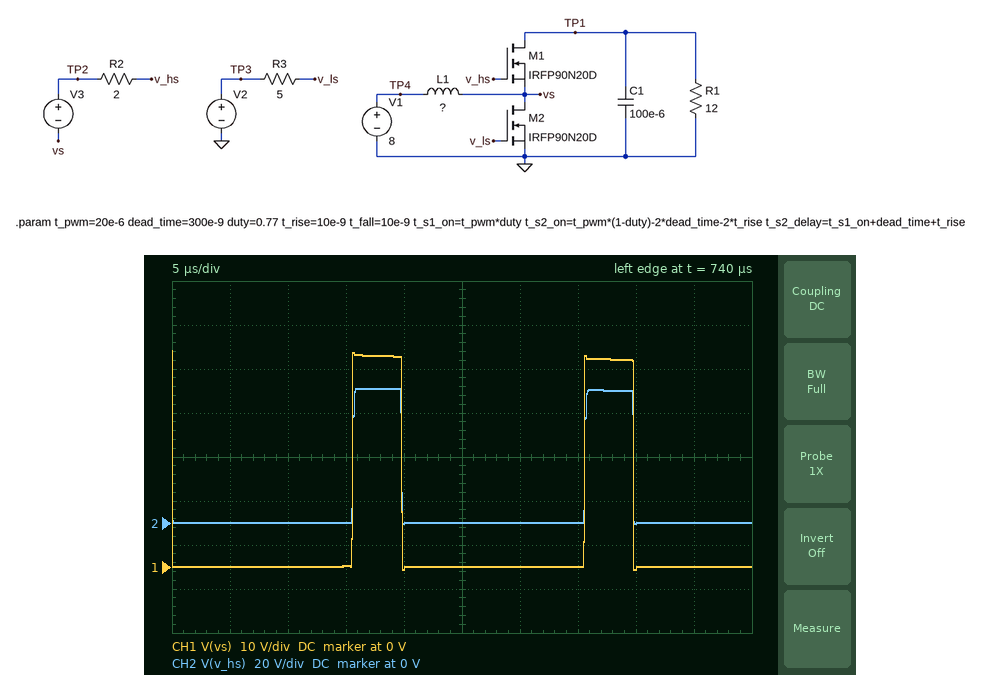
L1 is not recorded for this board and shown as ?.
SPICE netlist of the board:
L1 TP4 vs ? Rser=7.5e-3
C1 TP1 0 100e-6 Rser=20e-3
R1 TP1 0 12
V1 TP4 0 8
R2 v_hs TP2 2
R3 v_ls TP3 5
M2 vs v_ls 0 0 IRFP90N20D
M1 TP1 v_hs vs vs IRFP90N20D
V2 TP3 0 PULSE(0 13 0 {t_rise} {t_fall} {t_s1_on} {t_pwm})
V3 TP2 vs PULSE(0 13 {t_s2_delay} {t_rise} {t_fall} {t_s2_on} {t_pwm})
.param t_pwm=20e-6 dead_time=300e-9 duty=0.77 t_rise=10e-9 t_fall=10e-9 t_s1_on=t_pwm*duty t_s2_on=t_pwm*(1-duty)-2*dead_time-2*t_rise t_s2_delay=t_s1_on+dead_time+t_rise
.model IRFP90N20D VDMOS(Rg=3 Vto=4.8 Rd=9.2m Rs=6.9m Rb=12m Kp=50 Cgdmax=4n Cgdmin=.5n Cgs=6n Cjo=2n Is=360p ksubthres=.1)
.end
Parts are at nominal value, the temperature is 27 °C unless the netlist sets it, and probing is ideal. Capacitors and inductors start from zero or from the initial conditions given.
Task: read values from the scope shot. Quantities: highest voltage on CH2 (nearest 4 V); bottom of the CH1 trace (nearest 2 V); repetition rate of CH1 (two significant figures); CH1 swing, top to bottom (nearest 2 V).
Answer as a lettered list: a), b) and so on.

a) 60 V
b) 0 V
c) 50 kHz
d) 50 V
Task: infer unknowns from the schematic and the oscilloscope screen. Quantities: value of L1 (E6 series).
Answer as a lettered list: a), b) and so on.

a) 22 µH
